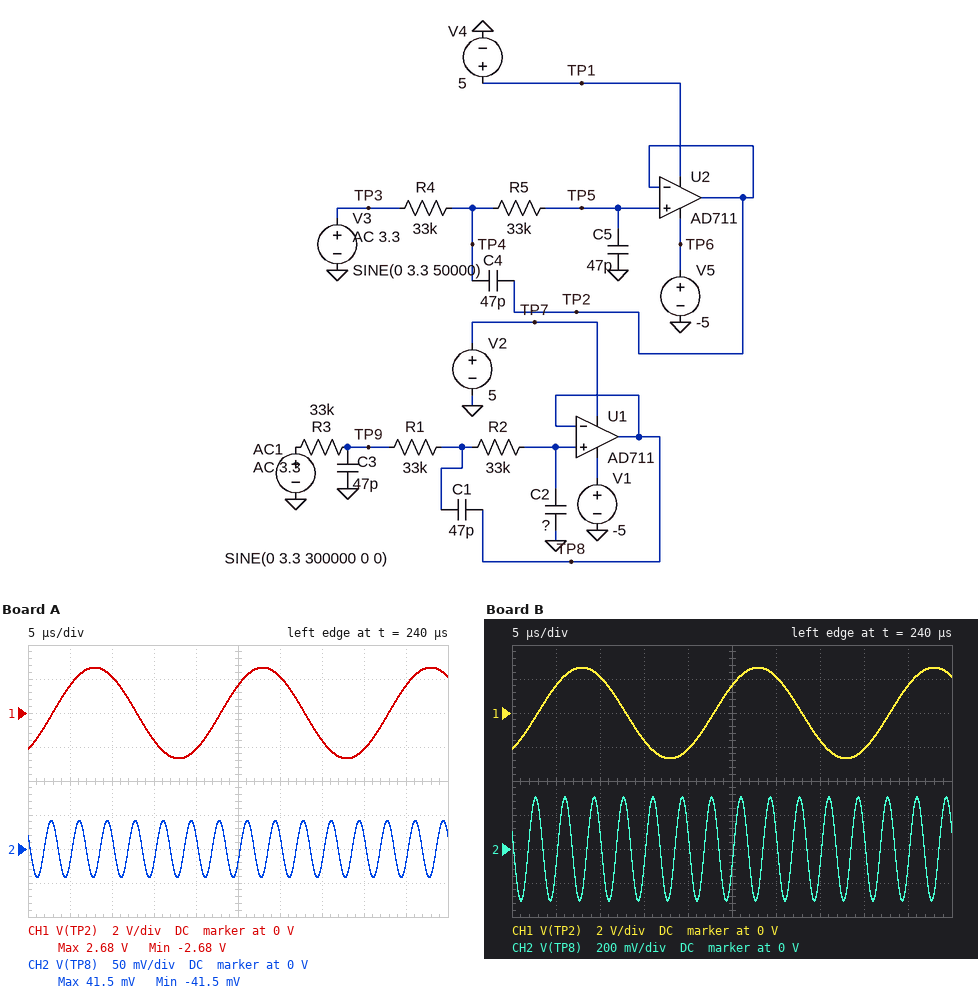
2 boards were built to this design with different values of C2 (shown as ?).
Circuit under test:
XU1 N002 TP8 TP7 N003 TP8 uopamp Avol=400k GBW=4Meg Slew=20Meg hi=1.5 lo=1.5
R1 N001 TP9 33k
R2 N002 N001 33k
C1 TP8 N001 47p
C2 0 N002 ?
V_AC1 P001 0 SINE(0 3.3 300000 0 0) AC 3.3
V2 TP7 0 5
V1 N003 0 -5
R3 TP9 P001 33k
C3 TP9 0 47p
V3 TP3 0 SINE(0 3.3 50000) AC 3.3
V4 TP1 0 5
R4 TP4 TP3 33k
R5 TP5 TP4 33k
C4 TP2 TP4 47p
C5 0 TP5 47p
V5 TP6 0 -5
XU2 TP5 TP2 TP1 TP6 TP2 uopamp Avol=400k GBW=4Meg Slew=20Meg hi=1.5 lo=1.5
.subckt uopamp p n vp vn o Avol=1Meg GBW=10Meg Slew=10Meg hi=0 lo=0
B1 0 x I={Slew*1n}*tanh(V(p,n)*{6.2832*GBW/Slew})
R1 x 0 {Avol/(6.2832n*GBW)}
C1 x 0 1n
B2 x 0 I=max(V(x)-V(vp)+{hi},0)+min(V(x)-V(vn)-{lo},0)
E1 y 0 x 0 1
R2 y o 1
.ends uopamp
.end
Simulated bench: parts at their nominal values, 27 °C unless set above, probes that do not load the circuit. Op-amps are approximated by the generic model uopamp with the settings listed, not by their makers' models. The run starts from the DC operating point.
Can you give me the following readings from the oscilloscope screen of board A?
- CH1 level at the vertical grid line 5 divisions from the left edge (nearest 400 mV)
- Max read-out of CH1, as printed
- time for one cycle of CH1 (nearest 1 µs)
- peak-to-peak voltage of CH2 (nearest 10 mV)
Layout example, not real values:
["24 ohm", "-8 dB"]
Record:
["1.6 V", "2.68 V", "20 µs", "80 mV"]
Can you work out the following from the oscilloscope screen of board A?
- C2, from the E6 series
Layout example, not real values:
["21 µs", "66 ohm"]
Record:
["100 pF"]
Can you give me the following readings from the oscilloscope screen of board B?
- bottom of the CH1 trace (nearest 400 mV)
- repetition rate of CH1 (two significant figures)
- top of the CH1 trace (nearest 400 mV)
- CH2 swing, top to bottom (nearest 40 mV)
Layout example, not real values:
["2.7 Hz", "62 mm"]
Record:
["-2.8 V", "50 kHz", "2.8 V", "600 mV"]
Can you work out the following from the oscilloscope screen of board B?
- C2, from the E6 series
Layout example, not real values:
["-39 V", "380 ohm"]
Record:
["15 pF"]
